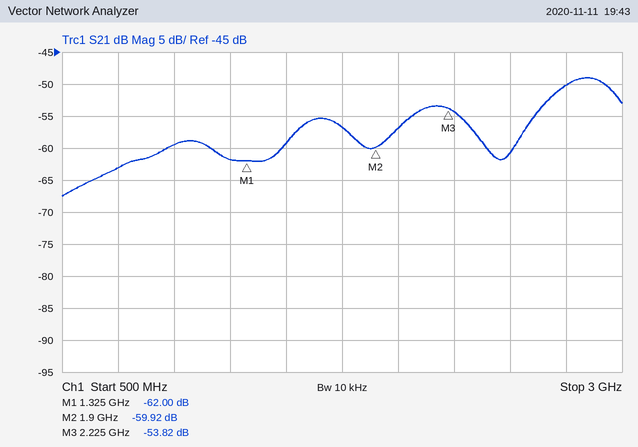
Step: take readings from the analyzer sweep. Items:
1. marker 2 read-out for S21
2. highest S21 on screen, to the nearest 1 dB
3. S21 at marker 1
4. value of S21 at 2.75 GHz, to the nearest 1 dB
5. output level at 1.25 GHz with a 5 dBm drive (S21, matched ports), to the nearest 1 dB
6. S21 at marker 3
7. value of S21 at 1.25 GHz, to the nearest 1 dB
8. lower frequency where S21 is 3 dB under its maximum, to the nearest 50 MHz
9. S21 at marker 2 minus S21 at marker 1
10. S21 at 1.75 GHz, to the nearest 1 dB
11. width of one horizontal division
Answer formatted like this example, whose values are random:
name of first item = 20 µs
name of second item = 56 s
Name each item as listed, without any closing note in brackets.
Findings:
marker 2 read-out for S21 = -59.92 dB
highest S21 on screen, to the nearest 1 dB = -49 dB
S21 at marker 1 = -62.00 dB
value of S21 at 2.75 GHz, to the nearest 1 dB = -50 dB
output level at 1.25 GHz with a 5 dBm drive (S21, matched ports), to the nearest 1 dB = -57 dBm
S21 at marker 3 = -53.82 dB
value of S21 at 1.25 GHz, to the nearest 1 dB = -62 dB
lower frequency where S21 is 3 dB under its maximum, to the nearest 50 MHz = 2.70 GHz
S21 at marker 2 minus S21 at marker 1 = 2.08 dB
S21 at 1.75 GHz, to the nearest 1 dB = -57 dB
width of one horizontal division = 250 MHz
